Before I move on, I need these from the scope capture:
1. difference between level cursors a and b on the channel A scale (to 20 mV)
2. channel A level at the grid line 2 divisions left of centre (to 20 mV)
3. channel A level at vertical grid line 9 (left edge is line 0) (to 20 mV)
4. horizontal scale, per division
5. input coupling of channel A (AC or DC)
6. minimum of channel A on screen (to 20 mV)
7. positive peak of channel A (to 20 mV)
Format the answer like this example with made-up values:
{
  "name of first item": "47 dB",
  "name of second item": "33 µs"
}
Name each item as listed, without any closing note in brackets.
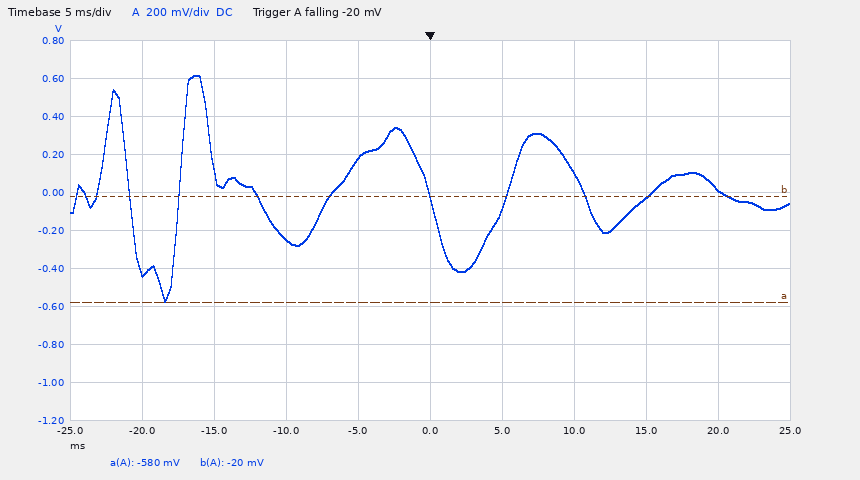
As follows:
{
  "difference between level cursors a and b on the channel A scale": "560 mV",
  "channel A level at the grid line 2 divisions left of centre": "-240 mV",
  "channel A level at vertical grid line 9 (left edge is line 0)": "20 mV",
  "horizontal scale, per division": "5 ms",
  "input coupling of channel A": "DC",
  "minimum of channel A on screen": "-580 mV",
  "positive peak of channel A": "620 mV"
}
